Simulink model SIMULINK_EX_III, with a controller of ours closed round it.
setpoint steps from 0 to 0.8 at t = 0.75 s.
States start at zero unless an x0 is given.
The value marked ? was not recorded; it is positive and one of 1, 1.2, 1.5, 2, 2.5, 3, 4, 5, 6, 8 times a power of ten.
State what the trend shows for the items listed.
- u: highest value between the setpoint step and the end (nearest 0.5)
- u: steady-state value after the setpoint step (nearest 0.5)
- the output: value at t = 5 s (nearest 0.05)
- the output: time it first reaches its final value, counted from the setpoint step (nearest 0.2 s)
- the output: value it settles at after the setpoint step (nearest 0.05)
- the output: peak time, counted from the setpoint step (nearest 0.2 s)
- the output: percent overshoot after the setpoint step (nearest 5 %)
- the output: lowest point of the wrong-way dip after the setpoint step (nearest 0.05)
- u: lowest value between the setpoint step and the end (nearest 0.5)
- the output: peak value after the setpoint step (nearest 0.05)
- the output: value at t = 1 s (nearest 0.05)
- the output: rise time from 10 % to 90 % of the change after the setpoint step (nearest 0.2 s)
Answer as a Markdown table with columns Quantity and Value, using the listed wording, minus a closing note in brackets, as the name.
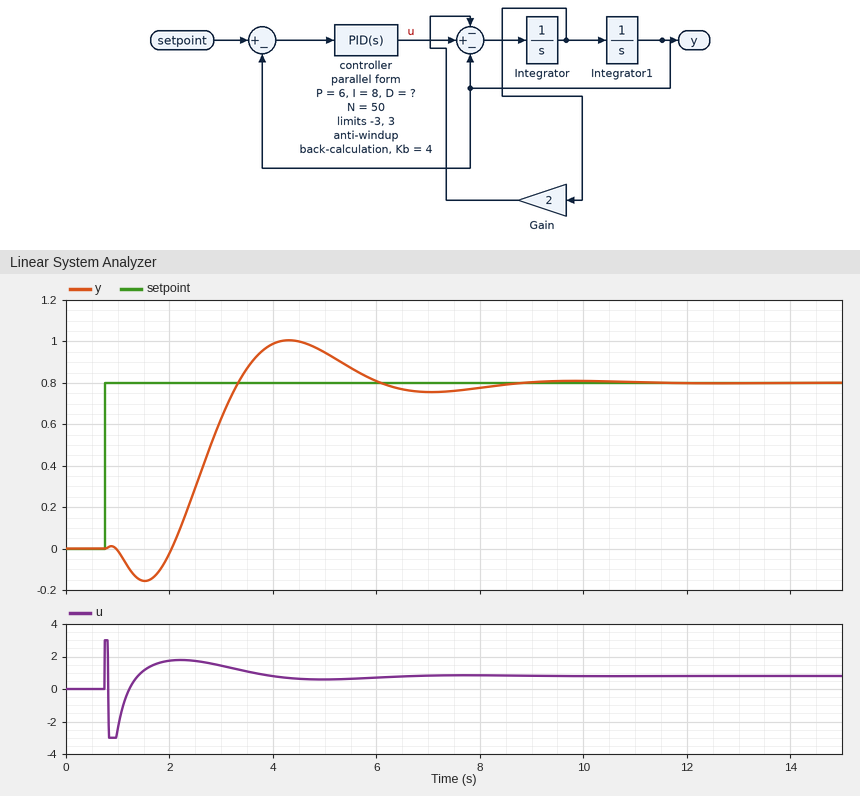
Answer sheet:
| Quantity | Value |
|---|---|
| u: highest value between the setpoint step and the end | 3.0 |
| u: steady-state value after the setpoint step | 1.0 |
| the output: value at t = 5 s | 0.95 |
| the output: time it first reaches its final value, counted from the setpoint step | 2.6 s |
| the output: value it settles at after the setpoint step | 0.80 |
| the output: peak time, counted from the setpoint step | 3.6 s |
| the output: percent overshoot after the setpoint step | 25 % |
| the output: lowest point of the wrong-way dip after the setpoint step | -0.15 |
| u: lowest value between the setpoint step and the end | -3.0 |
| the output: peak value after the setpoint step | 1.00 |
| the output: value at t = 1 s | 0.00 |
| the output: rise time from 10 % to 90 % of the change after the setpoint step | 1.0 s |
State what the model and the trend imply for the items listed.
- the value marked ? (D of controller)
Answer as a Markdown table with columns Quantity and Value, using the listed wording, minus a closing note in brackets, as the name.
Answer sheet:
| Quantity | Value |
|---|---|
| the value marked ? | 4 |
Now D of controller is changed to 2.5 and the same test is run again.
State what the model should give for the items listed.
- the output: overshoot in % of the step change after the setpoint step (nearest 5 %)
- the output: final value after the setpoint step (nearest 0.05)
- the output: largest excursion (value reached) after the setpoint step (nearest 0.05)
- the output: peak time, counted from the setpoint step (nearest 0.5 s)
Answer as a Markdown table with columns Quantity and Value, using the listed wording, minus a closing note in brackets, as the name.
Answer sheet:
| Quantity | Value |
|---|---|
| the output: overshoot in % of the step change after the setpoint step | 15 % |
| the output: final value after the setpoint step | 0.80 |
| the output: largest excursion (value reached) after the setpoint step | 0.95 |
| the output: peak time, counted from the setpoint step | 3.0 s |
